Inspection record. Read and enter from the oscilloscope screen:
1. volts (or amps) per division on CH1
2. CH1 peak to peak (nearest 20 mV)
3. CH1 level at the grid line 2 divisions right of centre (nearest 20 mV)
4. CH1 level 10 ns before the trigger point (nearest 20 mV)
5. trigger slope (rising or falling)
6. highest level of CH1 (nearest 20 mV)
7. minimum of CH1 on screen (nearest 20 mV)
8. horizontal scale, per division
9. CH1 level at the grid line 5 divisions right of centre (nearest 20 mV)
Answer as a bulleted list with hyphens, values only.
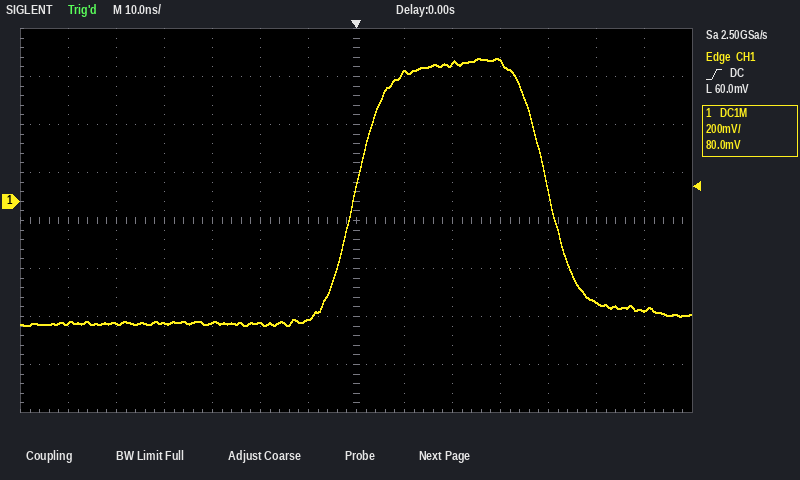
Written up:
- 200 mV
- 1.12 V
- 580 mV
- -500 mV
- rising
- 600 mV
- -520 mV
- 10 ns
- -420 mV
